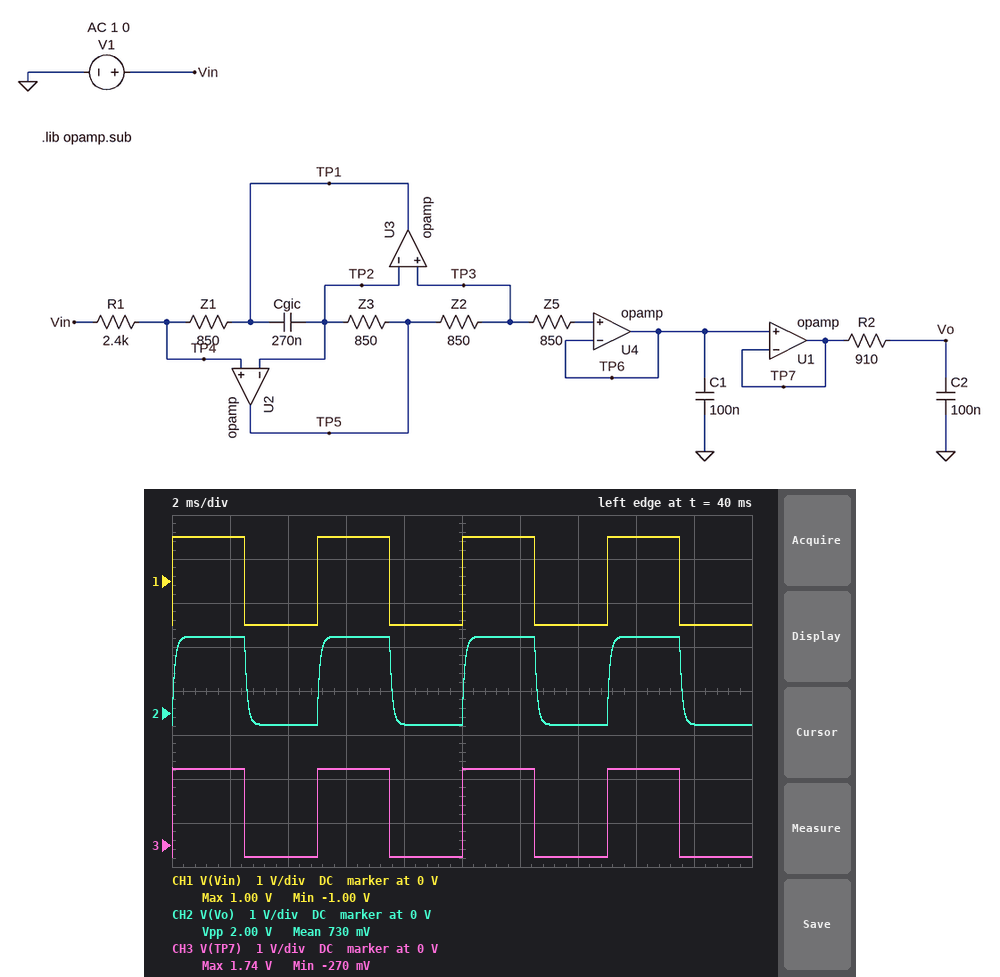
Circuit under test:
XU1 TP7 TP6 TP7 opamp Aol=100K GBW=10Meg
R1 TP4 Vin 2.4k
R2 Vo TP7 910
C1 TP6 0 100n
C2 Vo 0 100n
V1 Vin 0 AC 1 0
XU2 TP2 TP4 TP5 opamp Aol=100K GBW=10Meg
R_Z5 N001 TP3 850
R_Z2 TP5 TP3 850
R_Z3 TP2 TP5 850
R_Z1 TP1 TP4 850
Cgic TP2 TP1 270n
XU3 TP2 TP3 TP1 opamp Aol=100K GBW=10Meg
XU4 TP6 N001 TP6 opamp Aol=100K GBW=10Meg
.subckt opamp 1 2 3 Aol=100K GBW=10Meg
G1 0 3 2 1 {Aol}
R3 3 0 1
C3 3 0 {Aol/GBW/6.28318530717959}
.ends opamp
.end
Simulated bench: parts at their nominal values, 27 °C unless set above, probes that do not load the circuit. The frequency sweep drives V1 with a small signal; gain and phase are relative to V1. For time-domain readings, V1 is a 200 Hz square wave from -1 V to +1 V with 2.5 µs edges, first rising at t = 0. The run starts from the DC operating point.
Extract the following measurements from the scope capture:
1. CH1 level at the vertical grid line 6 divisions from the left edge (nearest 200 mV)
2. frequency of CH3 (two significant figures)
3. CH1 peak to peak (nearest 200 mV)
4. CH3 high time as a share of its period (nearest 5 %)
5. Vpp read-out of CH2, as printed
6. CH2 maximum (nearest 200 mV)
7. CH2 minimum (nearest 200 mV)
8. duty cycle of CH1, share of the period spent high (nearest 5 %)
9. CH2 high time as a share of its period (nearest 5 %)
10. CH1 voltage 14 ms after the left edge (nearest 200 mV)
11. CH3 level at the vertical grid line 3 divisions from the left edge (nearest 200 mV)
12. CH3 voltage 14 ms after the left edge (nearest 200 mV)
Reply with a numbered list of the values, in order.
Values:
1. 1.0 V
2. 200 Hz
3. 2.0 V
4. 50 %
5. 2.00 V
6. 1.8 V
7. -200 mV
8. 50 %
9. 50 %
10. -1.0 V
11. 1.8 V
12. -200 mV
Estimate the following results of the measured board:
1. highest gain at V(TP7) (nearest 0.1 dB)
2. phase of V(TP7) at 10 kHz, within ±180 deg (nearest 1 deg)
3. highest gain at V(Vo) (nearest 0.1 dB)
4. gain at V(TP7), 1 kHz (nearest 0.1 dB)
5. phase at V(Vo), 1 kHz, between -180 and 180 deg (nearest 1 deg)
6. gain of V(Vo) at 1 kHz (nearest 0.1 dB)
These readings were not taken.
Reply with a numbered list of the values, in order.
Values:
1. 0 dB
2. 0 deg
3. 0 dB
4. 0 dB
5. -30 deg
6. -1.2 dB
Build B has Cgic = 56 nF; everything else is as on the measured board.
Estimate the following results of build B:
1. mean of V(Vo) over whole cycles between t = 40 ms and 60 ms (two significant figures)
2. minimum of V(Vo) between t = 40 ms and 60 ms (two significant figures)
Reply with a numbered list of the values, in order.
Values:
1. 710 mV
2. -300 mV
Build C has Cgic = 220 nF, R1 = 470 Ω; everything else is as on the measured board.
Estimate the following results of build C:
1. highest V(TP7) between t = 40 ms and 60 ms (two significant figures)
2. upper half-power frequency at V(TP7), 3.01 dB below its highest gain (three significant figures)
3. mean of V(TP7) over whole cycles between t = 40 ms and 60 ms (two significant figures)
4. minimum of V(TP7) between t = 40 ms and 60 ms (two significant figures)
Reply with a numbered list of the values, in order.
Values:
1. 1.4 V
2. 7.27 MHz
3. 350 mV
4. -650 mV
